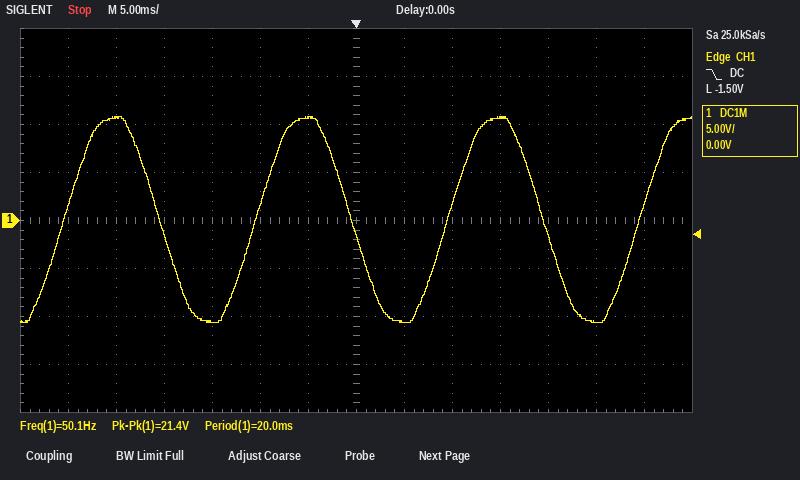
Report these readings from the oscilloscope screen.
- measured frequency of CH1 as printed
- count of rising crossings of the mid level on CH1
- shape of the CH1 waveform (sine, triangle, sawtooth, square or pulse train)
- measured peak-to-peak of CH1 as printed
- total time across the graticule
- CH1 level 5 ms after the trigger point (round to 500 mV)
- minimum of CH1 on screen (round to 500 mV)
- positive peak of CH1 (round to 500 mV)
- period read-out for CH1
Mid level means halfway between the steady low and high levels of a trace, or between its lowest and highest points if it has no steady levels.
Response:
50.1 Hz
4
sine
21.4 V
70 ms
-10.5 V
-10.5 V
11.0 V
20.0 ms
